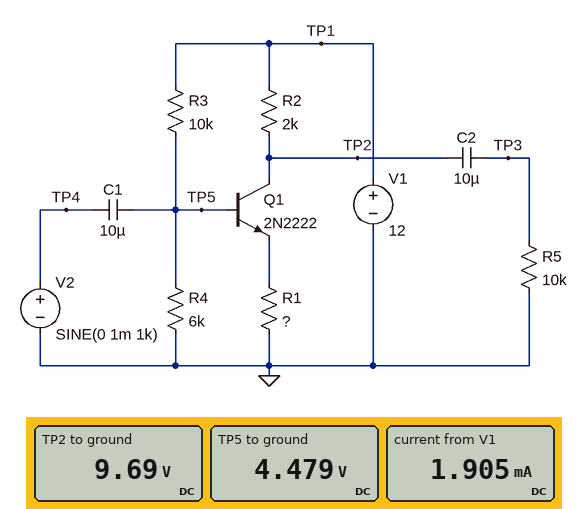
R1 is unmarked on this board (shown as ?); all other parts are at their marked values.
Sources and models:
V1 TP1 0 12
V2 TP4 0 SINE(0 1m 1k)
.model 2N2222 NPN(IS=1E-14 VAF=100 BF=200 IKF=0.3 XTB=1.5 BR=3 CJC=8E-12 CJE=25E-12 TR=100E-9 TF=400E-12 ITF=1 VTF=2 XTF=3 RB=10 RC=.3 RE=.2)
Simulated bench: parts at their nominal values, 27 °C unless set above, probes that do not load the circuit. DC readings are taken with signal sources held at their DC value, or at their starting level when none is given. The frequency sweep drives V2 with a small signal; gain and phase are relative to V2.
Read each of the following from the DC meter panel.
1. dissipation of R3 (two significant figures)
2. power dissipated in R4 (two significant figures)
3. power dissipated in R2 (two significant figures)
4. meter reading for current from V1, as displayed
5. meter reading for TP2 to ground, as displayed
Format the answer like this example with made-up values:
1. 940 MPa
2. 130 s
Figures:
1. 5.7 mW
2. 3.3 mW
3. 2.7 mW
4. 1.905 mA
5. 9.69 V
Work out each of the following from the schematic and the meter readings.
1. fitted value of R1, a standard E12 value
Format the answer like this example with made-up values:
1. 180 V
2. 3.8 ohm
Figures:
1. 3.3 kΩ
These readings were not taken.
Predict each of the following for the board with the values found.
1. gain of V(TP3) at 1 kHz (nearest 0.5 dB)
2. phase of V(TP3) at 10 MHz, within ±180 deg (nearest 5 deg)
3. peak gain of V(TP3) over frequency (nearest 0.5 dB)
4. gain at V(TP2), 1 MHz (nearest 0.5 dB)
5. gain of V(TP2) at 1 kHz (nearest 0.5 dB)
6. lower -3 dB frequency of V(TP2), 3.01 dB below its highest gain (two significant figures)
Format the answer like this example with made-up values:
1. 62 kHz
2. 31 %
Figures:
1. -6.0 dB
2. 115 deg
3. 0 dB
4. -6.0 dB
5. -6.0 dB
6. 15 MHz
